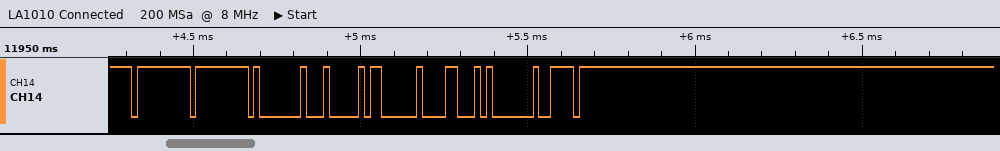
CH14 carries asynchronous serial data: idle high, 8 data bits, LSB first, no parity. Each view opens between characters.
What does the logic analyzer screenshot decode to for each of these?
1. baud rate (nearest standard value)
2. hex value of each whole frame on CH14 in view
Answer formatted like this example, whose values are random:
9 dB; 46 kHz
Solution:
57600 baud; FF, FF, 01, 04, 03, 18, 01, DE
